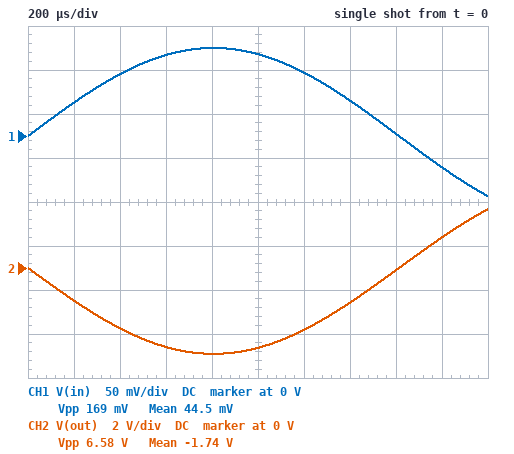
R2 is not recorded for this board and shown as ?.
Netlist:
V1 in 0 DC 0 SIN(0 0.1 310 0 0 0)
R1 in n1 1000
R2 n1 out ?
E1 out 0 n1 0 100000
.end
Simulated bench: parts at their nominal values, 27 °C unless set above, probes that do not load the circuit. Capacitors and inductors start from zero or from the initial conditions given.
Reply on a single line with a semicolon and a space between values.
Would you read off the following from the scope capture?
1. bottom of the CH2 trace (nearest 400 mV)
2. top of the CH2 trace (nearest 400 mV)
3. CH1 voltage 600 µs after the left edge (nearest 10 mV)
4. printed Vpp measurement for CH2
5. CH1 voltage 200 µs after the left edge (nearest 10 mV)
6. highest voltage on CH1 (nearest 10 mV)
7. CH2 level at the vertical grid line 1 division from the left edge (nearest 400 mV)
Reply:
-4.0 V; 2.8 V; 90 mV; 6.58 V; 40 mV; 100 mV; -1.6 V
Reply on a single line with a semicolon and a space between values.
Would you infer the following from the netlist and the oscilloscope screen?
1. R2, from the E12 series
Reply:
39 kΩ
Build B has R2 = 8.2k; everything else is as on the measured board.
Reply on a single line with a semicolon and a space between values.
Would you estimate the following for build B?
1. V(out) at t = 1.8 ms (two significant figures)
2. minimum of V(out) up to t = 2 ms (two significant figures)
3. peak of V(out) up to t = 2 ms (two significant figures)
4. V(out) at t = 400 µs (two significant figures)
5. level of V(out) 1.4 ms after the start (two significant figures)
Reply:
290 mV; -820 mV; 560 mV; -580 mV; -330 mV
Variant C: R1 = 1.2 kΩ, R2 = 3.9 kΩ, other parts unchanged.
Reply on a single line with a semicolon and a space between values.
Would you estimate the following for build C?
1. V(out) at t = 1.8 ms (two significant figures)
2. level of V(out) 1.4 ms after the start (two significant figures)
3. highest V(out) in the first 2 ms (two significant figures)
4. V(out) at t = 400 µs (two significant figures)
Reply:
120 mV; -130 mV; 220 mV; -230 mV
